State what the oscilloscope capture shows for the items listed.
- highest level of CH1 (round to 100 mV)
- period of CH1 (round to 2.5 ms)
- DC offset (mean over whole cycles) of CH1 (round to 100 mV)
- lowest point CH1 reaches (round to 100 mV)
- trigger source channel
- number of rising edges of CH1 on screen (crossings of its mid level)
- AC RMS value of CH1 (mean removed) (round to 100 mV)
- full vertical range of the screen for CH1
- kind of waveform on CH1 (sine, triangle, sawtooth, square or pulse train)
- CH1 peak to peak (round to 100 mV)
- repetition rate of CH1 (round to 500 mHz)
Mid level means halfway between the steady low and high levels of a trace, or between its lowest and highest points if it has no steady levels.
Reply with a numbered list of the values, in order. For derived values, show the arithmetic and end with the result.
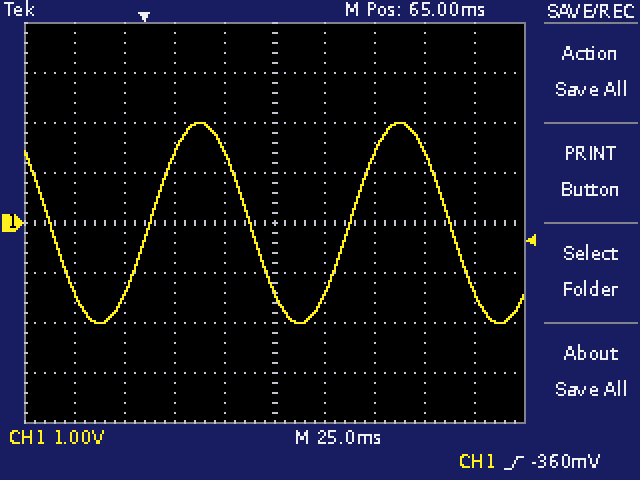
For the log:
1. 2.0 V
2. 100.0 ms
3. (2.0 V + (-2.0 V)) / 2 ≈ 0.0 V
4. -2.0 V
5. CH1
6. 2
7. 4.0 V / (2√2) ≈ 1.4 V
8. 8 V
9. sine
10. 2.0 V − (-2.0 V) = 4.0 V
11. 1 / 100.0 ms ≈ 10.0 Hz
